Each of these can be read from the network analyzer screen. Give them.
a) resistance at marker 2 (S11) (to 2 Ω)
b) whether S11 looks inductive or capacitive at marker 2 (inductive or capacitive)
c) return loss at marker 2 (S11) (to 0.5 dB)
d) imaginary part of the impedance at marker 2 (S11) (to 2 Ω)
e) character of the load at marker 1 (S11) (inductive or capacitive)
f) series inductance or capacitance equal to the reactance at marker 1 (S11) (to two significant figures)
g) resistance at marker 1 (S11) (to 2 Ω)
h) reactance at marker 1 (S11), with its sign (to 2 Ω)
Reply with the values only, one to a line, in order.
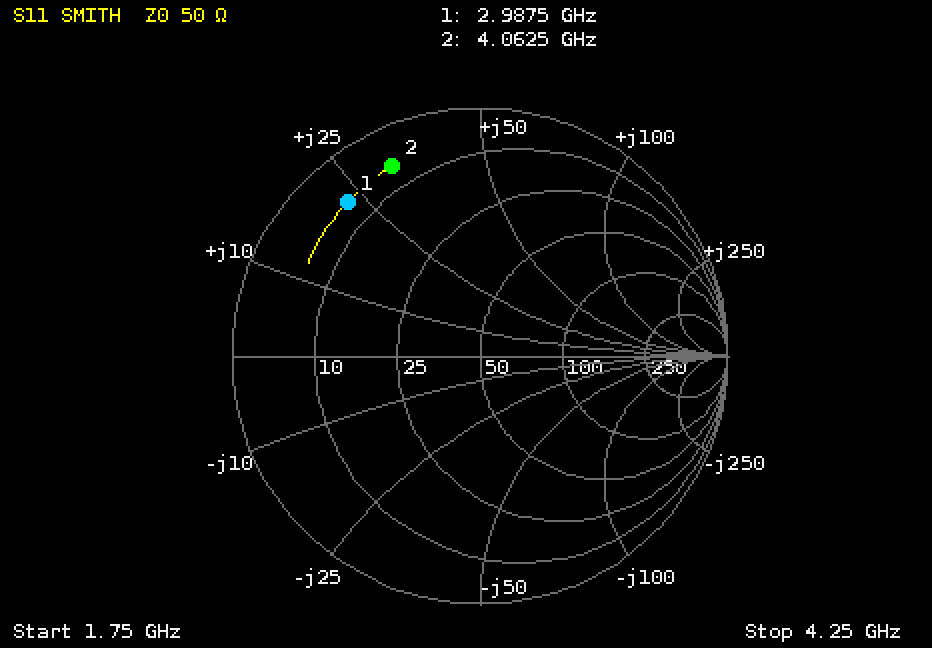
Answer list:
6 Ω
inductive
1.5 dB
+32 Ω
inductive
1.2 nH
6 Ω
+22 Ω
